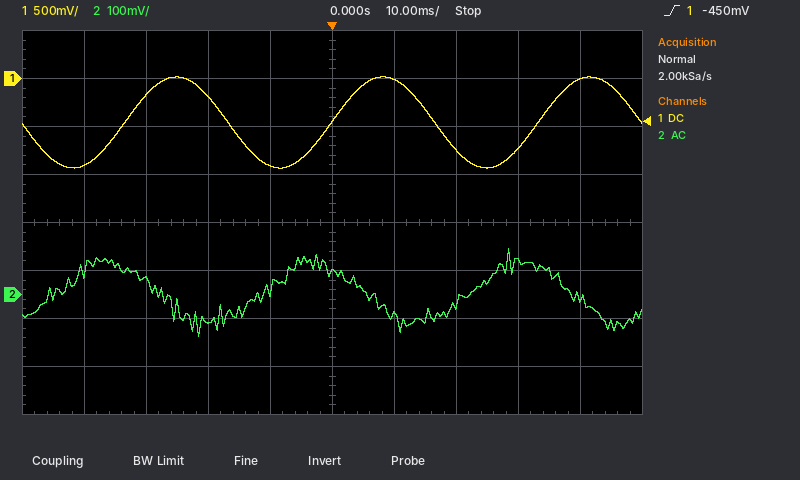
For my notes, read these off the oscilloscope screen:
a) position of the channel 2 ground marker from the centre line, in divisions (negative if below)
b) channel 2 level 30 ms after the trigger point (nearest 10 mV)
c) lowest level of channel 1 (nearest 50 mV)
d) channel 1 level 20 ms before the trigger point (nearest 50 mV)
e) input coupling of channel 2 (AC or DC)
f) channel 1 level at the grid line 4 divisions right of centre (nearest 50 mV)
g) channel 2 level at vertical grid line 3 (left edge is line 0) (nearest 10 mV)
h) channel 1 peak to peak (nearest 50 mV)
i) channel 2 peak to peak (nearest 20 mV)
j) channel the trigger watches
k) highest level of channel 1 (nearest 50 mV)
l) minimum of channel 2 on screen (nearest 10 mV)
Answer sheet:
-1.5 div
70 mV
-950 mV
-200 mV
AC
0 mV
-60 mV
950 mV
180 mV
channel 1
0 mV
-90 mV
